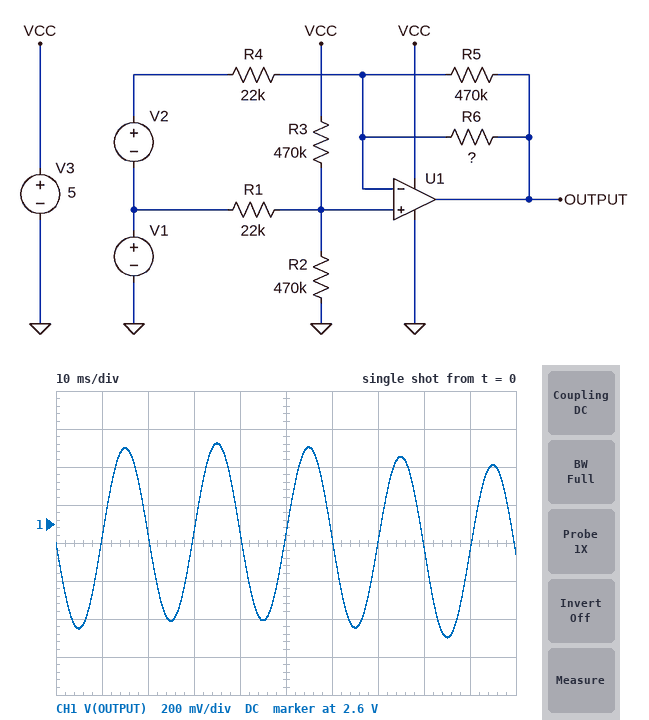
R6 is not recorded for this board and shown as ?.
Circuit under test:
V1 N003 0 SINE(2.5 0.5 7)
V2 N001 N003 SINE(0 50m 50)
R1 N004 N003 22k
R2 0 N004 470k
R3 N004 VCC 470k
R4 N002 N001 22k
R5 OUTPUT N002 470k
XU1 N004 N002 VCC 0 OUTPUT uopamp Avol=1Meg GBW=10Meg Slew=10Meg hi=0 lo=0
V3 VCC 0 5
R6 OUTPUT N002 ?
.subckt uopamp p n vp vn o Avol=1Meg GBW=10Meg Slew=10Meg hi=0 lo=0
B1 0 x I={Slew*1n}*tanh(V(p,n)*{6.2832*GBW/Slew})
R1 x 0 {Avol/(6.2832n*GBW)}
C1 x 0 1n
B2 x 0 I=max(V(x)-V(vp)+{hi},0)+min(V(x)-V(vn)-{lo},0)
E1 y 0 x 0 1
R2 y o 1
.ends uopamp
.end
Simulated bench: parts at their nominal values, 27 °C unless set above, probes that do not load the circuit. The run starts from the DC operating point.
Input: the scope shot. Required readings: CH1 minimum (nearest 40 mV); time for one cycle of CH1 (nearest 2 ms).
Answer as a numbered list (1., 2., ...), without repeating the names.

1. 2.00 V
2. 20 ms
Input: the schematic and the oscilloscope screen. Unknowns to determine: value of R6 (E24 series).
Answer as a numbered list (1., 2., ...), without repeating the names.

1. 360 kΩ
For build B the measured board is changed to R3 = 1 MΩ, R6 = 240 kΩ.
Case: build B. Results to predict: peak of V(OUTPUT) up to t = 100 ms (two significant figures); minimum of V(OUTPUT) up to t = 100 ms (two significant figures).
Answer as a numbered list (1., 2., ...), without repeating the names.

1. 2.6 V
2. 1.5 V
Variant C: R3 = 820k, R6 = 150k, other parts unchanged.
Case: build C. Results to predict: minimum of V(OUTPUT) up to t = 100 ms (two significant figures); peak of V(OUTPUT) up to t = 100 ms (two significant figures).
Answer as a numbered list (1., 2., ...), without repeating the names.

1. 1.8 V
2. 2.8 V
